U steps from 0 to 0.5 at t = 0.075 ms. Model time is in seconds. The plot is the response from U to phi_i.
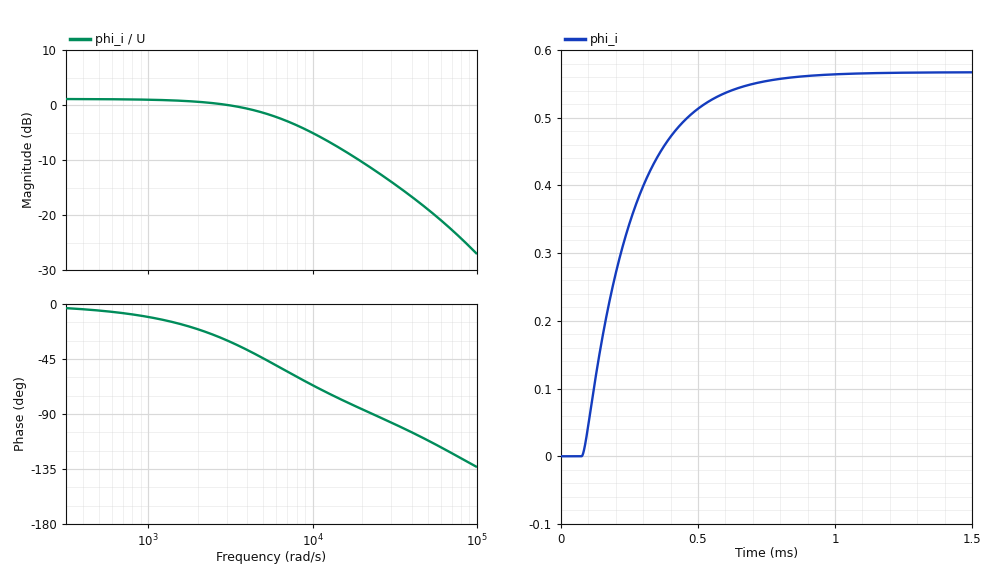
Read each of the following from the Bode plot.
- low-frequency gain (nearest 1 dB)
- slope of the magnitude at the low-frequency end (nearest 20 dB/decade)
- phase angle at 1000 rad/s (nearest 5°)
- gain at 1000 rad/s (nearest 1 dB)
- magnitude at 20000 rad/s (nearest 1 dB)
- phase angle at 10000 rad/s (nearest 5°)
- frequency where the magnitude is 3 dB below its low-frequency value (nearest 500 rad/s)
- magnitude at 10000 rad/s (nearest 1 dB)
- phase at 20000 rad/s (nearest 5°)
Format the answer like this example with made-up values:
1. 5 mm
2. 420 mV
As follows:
1. 1 dB
2. 0 dB/decade
3. -10°
4. 1 dB
5. -10 dB
6. -65°
7. 5500 rad/s
8. -5 dB
9. -85°
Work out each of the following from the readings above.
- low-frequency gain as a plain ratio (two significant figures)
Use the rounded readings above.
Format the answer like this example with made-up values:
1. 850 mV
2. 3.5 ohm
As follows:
1. 1.1
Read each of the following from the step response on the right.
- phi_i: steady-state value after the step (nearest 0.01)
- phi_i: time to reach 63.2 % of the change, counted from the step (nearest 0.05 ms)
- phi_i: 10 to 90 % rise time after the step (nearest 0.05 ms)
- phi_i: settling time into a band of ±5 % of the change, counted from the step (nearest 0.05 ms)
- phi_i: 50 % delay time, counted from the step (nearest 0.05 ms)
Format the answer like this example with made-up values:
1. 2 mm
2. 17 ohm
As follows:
1. 0.57
2. 0.20 ms
3. 0.40 ms
4. 0.55 ms
5. 0.15 ms
